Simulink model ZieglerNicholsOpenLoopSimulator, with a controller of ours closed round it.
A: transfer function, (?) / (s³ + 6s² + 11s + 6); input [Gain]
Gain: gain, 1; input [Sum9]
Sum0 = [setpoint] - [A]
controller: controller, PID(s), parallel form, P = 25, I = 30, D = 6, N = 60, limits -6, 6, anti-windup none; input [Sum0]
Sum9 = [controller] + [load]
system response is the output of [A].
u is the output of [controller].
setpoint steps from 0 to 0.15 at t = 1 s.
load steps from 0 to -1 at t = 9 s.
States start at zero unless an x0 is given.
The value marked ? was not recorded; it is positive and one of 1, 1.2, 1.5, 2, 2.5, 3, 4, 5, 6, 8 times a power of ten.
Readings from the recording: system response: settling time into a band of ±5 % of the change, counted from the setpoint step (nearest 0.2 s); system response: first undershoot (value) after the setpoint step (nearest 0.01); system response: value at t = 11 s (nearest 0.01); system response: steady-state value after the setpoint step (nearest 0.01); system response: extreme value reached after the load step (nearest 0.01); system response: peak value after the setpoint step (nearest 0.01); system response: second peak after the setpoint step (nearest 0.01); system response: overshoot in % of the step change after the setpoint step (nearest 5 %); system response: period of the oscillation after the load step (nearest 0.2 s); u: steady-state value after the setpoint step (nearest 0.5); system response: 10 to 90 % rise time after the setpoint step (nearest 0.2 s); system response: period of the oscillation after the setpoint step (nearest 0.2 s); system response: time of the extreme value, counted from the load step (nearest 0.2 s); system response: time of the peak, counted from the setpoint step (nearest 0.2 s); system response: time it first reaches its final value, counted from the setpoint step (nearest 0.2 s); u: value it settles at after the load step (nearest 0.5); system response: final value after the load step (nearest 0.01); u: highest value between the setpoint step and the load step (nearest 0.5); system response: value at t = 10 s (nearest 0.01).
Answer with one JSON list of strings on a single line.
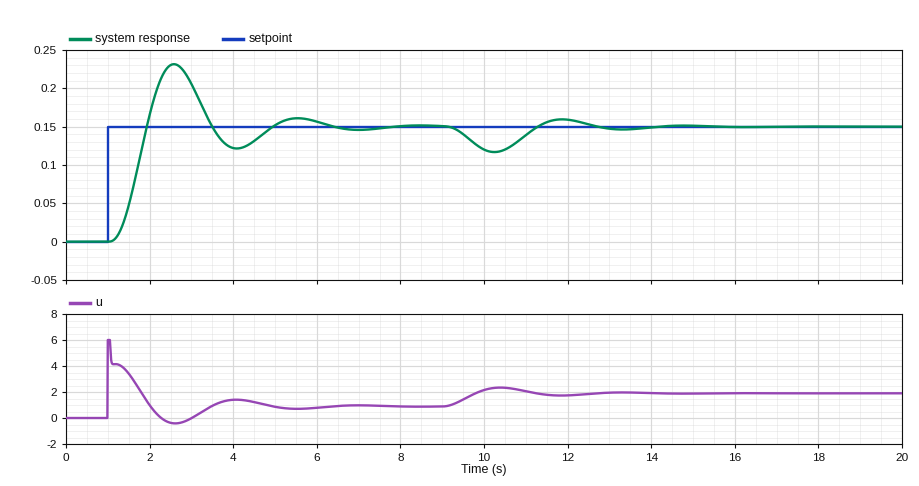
["5.0 s", "0.12", "0.14", "0.15", "0.12", "0.23", "0.16", "55 %", "3.0 s", "1.0", "0.6 s", "3.0 s", "1.2 s", "1.6 s", "1.0 s", "2.0", "0.15", "6.0", "0.12"]
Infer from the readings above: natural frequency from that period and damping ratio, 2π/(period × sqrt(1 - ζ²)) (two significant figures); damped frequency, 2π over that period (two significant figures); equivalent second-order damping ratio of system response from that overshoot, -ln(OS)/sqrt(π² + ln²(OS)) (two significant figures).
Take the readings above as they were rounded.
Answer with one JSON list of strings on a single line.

["2.1 rad/s", "2.1 rad/s", "0.19"]
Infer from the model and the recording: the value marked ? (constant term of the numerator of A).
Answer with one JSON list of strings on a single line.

["1"]
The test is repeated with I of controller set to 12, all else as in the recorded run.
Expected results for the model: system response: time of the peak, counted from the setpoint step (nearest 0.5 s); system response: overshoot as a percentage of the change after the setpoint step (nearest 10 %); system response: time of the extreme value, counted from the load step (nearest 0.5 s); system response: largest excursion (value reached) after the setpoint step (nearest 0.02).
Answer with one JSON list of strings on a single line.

["1.5 s", "20 %", "1.5 s", "0.18"]
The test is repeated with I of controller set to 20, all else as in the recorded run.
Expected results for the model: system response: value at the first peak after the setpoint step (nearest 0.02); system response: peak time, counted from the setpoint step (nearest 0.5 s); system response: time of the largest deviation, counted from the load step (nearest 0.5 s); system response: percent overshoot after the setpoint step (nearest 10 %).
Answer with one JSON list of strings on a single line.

["0.20", "1.5 s", "1.5 s", "40 %"]
